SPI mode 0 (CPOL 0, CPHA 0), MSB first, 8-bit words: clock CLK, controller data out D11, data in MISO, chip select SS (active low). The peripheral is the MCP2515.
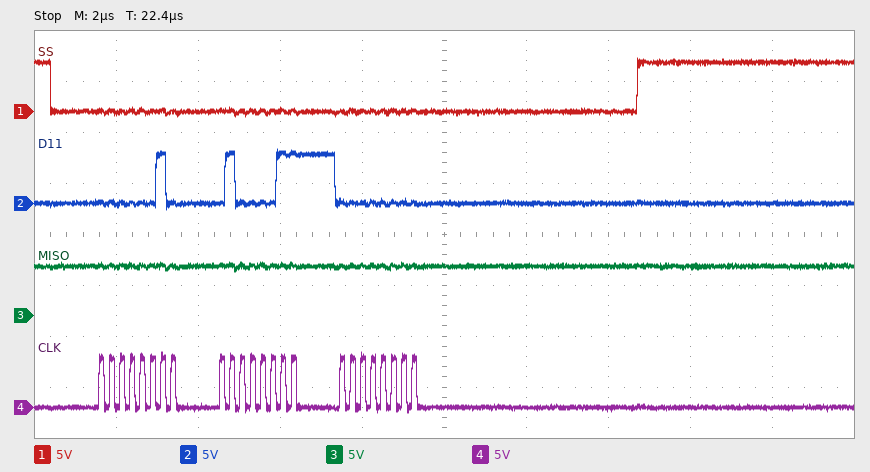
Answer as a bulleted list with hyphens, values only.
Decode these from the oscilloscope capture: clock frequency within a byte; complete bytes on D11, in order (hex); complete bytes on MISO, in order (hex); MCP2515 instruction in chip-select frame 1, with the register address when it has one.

- 4 MHz
- 02 43 00
- FF FF FF
- WRITE 0x43
